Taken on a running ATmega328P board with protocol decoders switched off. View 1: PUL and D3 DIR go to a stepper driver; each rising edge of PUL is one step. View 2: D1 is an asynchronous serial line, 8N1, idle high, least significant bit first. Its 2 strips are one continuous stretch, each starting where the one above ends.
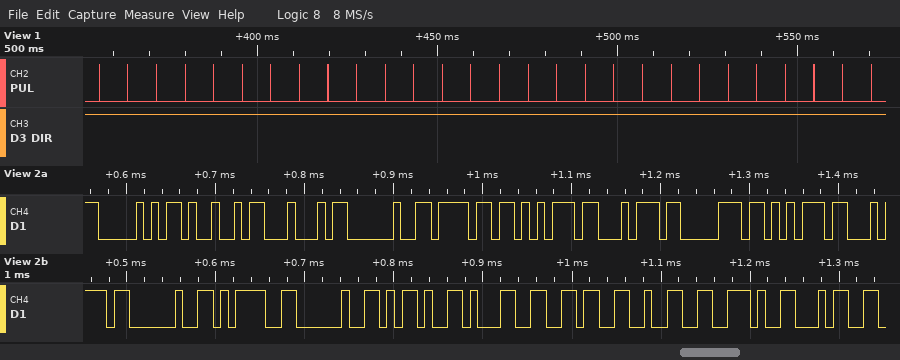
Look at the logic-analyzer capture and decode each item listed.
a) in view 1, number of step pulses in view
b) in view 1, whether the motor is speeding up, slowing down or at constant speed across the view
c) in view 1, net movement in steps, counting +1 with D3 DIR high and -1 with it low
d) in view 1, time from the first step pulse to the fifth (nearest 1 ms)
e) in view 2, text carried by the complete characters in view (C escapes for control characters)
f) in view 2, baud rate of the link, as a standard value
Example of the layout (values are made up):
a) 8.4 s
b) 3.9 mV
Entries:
a) 28
b) constant speed
c) +28
d) 32 ms
e) "PID output = -162.4"
f) 115200 baud
